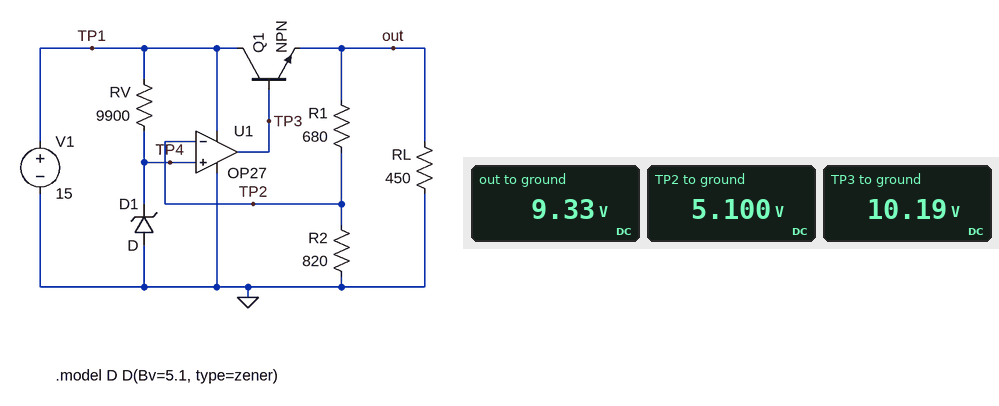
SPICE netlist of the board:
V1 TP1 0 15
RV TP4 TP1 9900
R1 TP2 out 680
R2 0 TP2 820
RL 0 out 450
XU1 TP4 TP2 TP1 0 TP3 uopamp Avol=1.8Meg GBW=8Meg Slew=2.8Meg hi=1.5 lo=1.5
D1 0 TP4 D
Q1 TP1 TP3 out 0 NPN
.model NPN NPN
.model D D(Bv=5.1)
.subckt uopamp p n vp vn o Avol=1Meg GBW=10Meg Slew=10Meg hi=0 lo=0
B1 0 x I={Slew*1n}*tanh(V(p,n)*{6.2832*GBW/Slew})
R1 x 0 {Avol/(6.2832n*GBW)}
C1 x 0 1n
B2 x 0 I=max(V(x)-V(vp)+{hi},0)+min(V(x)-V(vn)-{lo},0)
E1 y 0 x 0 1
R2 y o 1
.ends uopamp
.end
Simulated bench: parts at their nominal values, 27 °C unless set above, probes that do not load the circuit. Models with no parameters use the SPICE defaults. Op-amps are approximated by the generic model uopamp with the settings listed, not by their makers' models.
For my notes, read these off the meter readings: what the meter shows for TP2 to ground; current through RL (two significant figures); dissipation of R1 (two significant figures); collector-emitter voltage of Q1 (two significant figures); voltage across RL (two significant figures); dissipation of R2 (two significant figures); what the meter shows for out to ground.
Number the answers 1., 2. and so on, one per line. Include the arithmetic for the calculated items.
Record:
1. 5.100 V
2. (9.33 V) / 450 Ω = 21 mA
3. (9.33 V - 5.1 V)^2 / 680 Ω = 26 mW
4. 15 V - 9.33 V = 5.7 V
5. 9.33 V = 9.3 V
6. (5.1 V)^2 / 820 Ω = 32 mW
7. 9.33 V
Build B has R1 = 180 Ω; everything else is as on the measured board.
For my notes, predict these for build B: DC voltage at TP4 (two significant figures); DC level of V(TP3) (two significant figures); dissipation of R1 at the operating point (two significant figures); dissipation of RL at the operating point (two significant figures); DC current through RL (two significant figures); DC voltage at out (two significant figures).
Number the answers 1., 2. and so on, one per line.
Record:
1. 5.1 V
2. 7.1 V
3. 7.0 mW
4. 86 mW
5. 14 mA
6. 6.2 V
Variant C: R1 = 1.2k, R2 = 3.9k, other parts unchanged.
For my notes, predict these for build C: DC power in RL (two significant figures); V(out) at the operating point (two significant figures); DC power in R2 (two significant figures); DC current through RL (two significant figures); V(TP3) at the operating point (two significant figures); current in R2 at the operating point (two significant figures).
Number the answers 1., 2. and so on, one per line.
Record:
1. 99 mW
2. 6.7 V
3. 6.7 mW
4. 15 mA
5. 7.5 V
6. 1.3 mA
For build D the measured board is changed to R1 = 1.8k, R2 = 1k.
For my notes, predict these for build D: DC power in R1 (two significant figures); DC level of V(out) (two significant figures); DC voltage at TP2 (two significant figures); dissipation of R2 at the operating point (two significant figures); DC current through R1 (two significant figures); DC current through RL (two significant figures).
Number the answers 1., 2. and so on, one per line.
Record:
1. 37 mW
2. 13 V
3. 4.5 V
4. 20 mW
5. 4.5 mA
6. 28 mA
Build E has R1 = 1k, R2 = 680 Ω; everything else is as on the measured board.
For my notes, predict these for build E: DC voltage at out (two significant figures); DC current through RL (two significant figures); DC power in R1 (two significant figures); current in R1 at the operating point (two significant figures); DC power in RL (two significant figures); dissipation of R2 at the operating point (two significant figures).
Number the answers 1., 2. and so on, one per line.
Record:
1. 13 V
2. 28 mA
3. 56 mW
4. 7.5 mA
5. 350 mW
6. 38 mW
